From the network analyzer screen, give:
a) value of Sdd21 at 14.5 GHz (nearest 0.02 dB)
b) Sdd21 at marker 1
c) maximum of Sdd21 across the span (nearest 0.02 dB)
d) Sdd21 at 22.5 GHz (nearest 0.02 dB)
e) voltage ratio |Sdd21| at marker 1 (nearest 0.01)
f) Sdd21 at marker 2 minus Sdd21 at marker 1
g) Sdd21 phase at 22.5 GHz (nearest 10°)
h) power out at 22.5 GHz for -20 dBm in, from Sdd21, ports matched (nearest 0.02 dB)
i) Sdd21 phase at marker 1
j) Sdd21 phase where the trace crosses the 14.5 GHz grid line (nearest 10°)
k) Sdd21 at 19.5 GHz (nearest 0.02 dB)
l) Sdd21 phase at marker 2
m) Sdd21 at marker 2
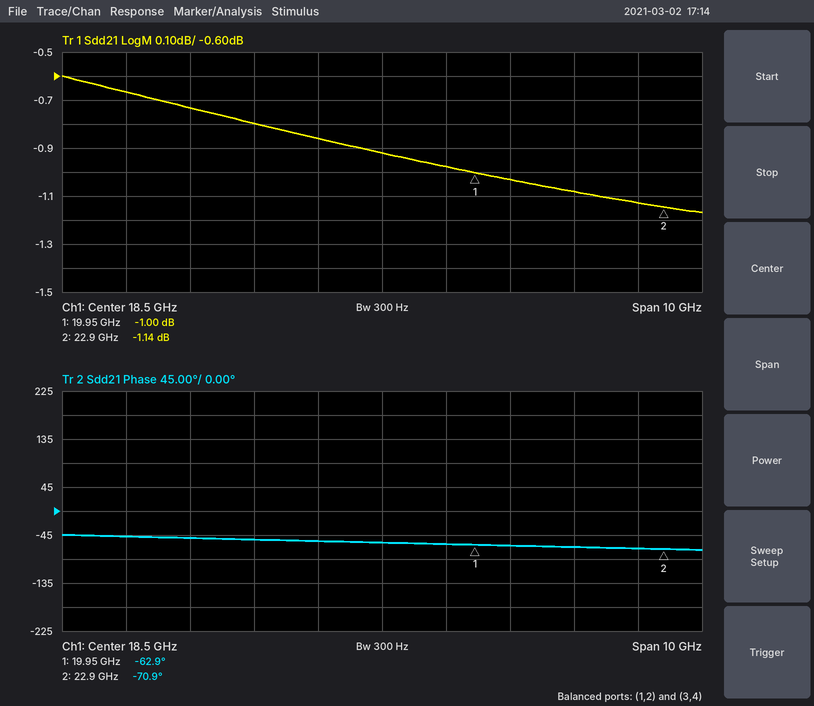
-0.66 dB
-1.00 dB
-0.60 dB
-1.12 dB
0.89
-0.14 dB
-70°
-21.12 dBm
-62.9°
-50°
-0.98 dB
-70.9°
-1.14 dB
